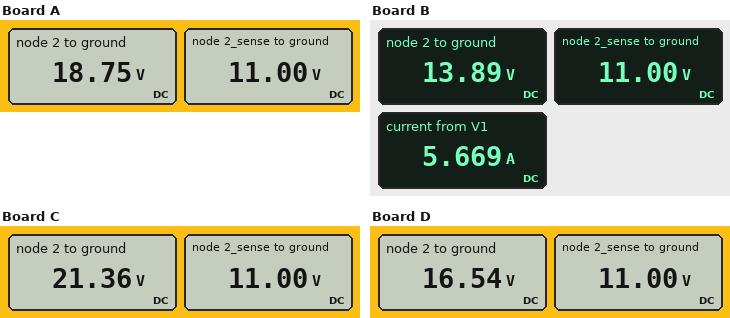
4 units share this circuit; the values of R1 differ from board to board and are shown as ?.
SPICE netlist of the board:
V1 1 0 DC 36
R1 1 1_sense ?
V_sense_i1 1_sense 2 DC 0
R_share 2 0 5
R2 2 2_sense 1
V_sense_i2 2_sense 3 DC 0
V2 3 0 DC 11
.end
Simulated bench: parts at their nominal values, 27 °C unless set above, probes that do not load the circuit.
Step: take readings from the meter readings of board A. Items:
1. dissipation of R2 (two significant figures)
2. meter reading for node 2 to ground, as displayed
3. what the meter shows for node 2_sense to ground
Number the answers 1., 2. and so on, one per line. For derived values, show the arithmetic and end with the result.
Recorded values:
1. (18.75 V - 11 V)^2 / 1 Ω = 60 W
2. 18.75 V
3. 11.00 V
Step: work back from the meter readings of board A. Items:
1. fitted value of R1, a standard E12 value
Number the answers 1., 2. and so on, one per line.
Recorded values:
1. 1.5 Ω
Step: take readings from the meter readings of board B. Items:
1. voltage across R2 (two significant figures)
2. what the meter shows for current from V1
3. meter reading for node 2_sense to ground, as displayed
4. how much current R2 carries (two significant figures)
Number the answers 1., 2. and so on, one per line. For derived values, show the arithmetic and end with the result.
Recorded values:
1. 13.89 V - 11 V = 2.9 V
2. 5.669 A
3. 11.00 V
4. (13.89 V - 11 V) / 1 Ω = 2.9 A
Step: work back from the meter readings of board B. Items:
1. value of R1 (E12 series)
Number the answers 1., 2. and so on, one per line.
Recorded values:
1. 3.9 Ω
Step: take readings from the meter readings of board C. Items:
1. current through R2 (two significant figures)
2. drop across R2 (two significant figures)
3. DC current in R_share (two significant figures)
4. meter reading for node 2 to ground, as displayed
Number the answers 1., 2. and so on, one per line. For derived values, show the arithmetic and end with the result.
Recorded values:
1. (21.36 V - 11 V) / 1 Ω = 10 A
2. 21.36 V - 11 V = 10 V
3. (21.36 V) / 5 Ω = 4.3 A
4. 21.36 V
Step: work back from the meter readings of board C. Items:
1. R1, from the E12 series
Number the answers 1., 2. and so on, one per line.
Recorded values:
1. 1 Ω
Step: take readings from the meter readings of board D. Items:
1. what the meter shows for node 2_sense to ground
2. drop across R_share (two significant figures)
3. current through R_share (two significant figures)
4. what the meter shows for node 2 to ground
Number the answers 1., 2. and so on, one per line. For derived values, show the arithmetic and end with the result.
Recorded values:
1. 11.00 V
2. 16.54 V = 17 V
3. (16.54 V) / 5 Ω = 3.3 A
4. 16.54 V
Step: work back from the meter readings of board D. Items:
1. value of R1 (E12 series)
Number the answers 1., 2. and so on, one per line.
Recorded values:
1. 2.2 Ω
